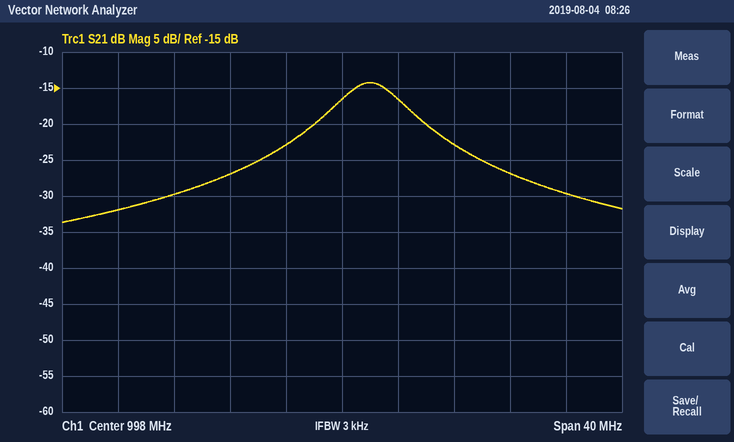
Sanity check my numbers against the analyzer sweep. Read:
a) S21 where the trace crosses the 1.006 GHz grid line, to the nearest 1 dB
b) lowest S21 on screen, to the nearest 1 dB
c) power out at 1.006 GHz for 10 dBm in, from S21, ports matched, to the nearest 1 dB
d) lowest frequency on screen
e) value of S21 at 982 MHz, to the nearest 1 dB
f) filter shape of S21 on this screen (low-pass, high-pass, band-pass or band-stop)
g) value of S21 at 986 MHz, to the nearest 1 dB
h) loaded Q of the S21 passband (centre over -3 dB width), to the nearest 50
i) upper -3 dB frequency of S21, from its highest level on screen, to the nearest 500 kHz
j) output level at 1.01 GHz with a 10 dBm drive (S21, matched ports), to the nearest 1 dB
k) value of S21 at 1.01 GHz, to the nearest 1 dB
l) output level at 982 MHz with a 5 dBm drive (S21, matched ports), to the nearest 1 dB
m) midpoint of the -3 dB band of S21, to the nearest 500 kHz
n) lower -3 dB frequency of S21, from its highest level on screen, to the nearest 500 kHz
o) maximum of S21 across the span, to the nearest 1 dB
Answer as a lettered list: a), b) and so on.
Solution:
a) -23 dB
b) -34 dB
c) -13 dBm
d) 978 MHz
e) -32 dB
f) band-pass
g) -30 dB
h) 200
i) 1.0025 GHz
j) -17 dBm
k) -27 dB
l) -27 dBm
m) 1.0000 GHz
n) 997.5 MHz
o) -14 dB
